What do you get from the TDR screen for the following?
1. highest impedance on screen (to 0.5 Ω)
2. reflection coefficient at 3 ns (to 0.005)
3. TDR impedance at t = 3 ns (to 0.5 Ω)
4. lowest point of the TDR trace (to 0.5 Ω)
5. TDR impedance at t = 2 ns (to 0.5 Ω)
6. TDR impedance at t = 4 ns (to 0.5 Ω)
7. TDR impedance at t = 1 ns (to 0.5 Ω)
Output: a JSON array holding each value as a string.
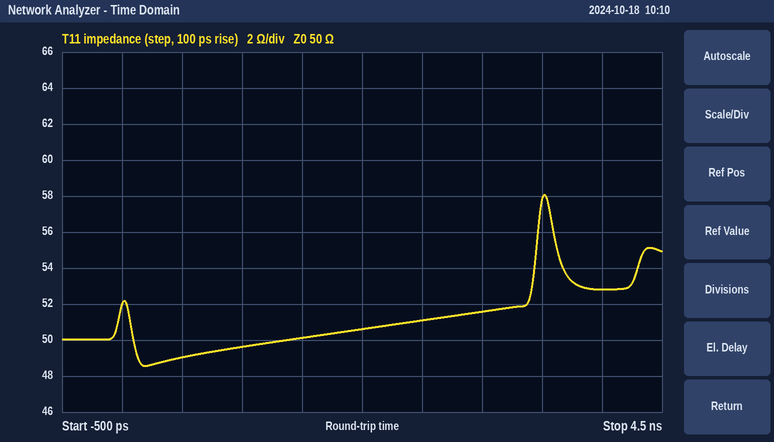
["58.0 Ω", "+0.015", "51.5 Ω", "48.5 Ω", "50.5 Ω", "53.0 Ω", "49.5 Ω"]
